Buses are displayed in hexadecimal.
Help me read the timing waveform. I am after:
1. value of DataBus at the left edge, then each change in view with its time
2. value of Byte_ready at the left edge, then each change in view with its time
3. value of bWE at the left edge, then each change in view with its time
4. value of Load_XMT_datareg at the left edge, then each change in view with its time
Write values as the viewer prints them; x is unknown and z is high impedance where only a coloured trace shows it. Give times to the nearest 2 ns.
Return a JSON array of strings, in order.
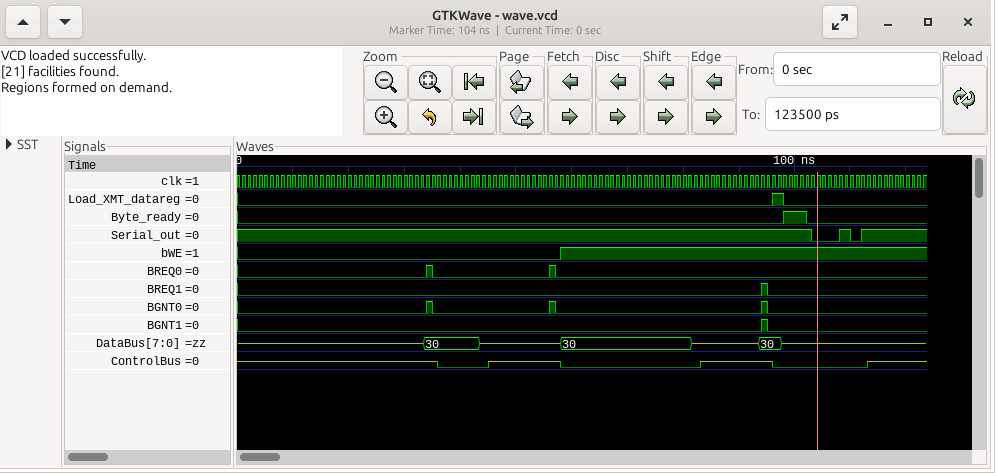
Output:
["z, 30 at 34 ns, z at 44 ns, 30 at 58 ns, z at 82 ns, 30 at 94 ns, z at 98 ns", "0, 1 at 98 ns, 0 at 102 ns", "0, 1 at 58 ns", "0, 1 at 96 ns, 0 at 98 ns"]
